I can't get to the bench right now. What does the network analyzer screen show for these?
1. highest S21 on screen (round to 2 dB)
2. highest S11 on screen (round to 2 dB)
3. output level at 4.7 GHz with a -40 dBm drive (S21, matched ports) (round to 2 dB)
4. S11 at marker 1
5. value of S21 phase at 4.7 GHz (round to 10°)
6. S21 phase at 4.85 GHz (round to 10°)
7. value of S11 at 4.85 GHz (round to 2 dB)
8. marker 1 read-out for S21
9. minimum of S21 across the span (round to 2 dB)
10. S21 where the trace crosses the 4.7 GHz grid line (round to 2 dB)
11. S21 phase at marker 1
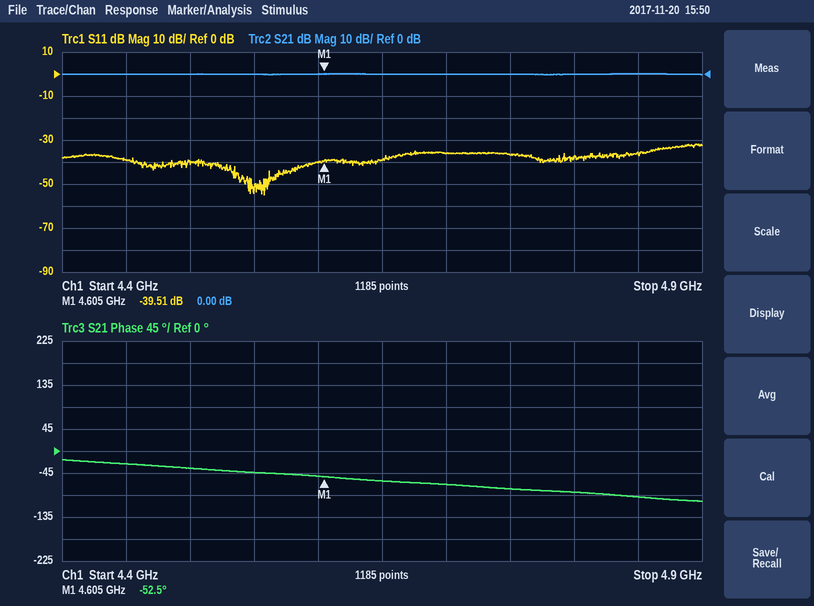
0 dB
-32 dB
-40 dBm
-39.51 dB
-70°
-90°
-36 dB
0.00 dB
0 dB
0 dB
-52.5°
